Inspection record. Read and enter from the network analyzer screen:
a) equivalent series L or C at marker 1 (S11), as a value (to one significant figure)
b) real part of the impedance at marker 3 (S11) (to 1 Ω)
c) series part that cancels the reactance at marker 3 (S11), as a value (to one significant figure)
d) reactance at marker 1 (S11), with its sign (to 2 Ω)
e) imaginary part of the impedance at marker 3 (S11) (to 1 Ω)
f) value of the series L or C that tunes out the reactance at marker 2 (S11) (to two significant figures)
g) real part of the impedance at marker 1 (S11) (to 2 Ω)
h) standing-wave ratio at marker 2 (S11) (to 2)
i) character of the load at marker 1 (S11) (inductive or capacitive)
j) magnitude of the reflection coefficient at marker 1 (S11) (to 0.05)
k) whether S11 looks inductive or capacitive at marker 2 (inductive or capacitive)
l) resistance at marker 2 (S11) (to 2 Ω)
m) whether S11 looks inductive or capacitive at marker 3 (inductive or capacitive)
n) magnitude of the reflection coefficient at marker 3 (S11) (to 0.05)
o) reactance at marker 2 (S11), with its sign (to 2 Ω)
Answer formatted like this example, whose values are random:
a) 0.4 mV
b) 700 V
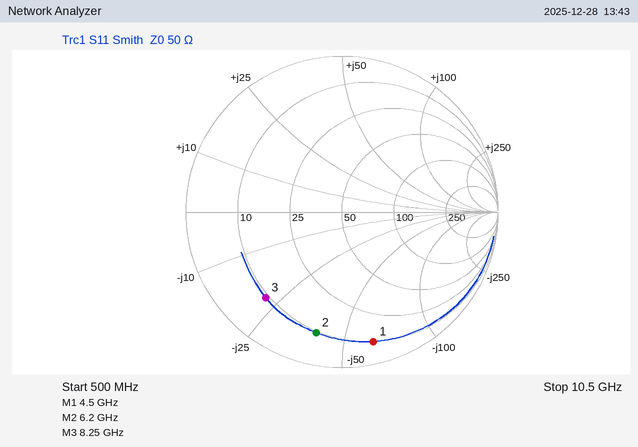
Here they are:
a) 600 fF
b) 9 Ω
c) 400 pH
d) -62 Ω
e) -22 Ω
f) 1.0 nH
g) 10 Ω
h) 8
i) capacitive
j) 0.85
k) capacitive
l) 10 Ω
m) capacitive
n) 0.75
o) -40 Ω
